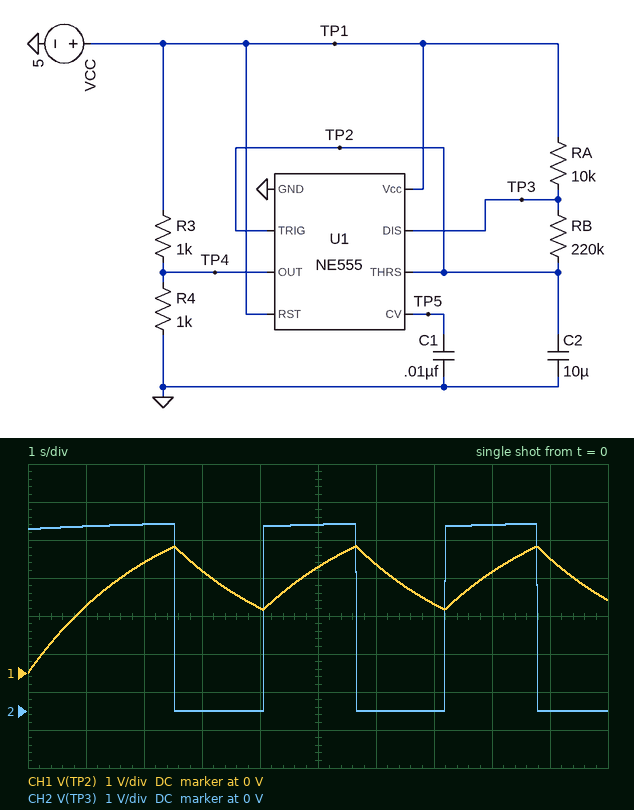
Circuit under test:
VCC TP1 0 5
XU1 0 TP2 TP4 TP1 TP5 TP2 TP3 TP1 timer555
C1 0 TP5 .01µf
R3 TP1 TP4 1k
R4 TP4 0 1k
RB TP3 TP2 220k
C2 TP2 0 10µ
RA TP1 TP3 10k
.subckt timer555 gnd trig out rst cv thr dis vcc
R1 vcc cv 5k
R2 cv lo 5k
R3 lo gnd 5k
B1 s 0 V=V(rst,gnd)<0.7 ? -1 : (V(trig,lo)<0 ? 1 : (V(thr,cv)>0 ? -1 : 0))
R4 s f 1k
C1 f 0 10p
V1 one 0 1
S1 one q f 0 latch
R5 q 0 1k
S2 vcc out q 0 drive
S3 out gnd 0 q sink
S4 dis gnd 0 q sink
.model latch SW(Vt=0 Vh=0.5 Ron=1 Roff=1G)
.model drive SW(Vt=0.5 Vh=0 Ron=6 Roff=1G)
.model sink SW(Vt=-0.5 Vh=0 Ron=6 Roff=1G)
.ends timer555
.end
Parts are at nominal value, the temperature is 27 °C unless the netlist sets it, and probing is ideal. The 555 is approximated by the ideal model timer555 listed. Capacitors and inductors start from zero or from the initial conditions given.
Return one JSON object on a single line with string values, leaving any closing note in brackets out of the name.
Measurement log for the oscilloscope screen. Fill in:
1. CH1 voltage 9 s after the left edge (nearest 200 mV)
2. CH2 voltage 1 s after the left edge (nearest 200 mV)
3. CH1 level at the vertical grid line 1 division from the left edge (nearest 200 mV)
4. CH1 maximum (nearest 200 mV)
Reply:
{"CH1 voltage 9 s after the left edge": "3.0 V", "CH2 voltage 1 s after the left edge": "4.8 V", "CH1 level at the vertical grid line 1 division from the left edge": "1.8 V", "CH1 maximum": "3.4 V"}
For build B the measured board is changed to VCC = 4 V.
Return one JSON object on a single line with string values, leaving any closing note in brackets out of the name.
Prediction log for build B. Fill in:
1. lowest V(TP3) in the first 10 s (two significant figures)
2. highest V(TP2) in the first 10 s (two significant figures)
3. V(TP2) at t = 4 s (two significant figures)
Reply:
{"lowest V(TP3) in the first 10 s": "2.4 mV", "highest V(TP2) in the first 10 s": "2.7 V", "V(TP2) at t = 4 s": "1.4 V"}
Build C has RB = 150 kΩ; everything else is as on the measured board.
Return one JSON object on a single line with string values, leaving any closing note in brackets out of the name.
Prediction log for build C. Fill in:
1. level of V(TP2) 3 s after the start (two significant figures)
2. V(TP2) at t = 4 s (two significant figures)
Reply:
{"level of V(TP2) 3 s after the start": "2.1 V", "V(TP2) at t = 4 s": "3.1 V"}
